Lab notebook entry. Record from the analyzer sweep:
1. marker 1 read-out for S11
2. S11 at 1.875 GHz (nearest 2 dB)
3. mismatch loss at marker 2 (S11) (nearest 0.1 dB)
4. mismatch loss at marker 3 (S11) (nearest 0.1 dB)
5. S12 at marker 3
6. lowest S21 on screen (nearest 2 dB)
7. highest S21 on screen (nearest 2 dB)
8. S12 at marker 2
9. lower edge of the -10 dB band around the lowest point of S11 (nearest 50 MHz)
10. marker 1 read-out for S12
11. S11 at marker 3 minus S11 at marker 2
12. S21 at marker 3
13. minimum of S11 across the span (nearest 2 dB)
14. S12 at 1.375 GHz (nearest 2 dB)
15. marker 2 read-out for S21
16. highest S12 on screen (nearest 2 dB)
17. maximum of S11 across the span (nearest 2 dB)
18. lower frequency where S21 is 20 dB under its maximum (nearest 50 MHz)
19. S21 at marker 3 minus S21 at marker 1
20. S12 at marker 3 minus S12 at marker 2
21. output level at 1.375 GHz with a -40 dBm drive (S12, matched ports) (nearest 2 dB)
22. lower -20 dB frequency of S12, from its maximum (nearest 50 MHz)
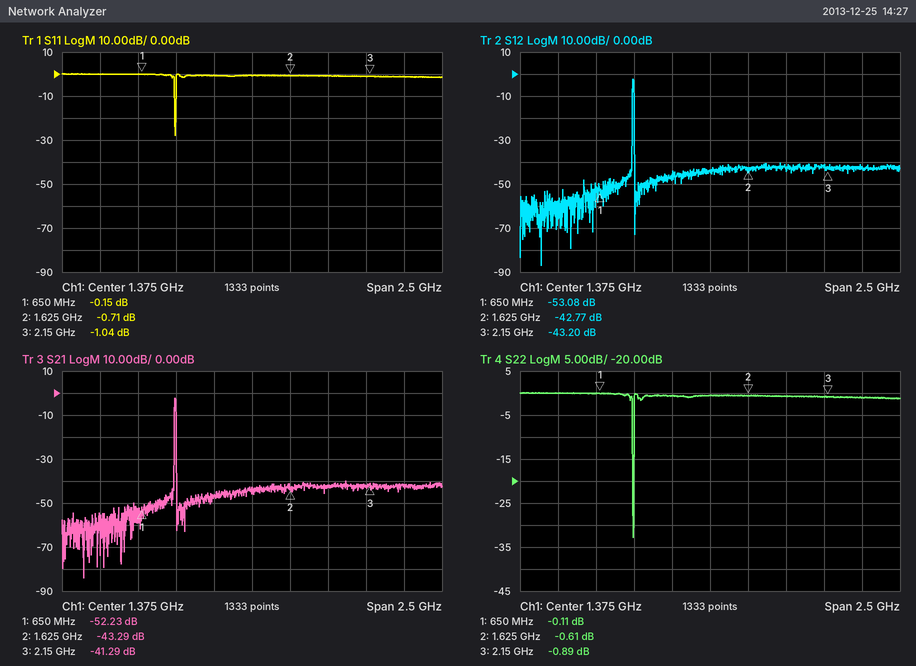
-0.15 dB
0 dB
8.2 dB
6.7 dB
-43.20 dB
-84 dB
-2 dB
-42.77 dB
850 MHz
-53.08 dB
-0.33 dB
-41.29 dB
-28 dB
-44 dB
-43.29 dB
-2 dB
0 dB
850 MHz
10.94 dB
-0.43 dB
-84 dBm
850 MHz
